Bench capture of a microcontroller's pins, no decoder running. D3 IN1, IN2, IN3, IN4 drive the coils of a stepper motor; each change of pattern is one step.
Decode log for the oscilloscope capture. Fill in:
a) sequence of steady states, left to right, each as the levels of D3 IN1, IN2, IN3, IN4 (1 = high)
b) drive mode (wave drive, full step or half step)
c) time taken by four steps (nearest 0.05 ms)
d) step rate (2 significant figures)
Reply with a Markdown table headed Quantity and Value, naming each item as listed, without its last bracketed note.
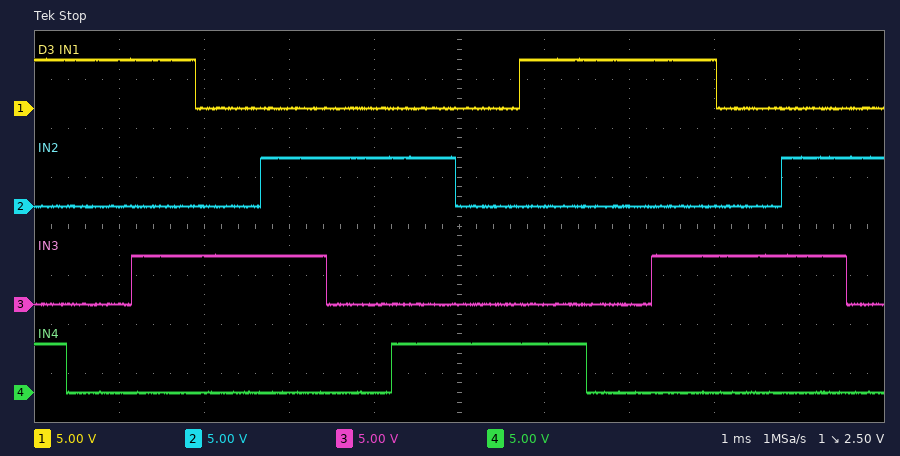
| Quantity | Value |
|---|---|
| sequence of steady states, left to right, each as the levels of D3 IN1, IN2, IN3, IN4 | 1001 1000 1010 0010 0110 0100 0101 0001 1001 1000 1010 0010 0110 0100 |
| drive mode | half step |
| time taken by four steps | 3.05 ms |
| step rate | 1300 steps/s |
